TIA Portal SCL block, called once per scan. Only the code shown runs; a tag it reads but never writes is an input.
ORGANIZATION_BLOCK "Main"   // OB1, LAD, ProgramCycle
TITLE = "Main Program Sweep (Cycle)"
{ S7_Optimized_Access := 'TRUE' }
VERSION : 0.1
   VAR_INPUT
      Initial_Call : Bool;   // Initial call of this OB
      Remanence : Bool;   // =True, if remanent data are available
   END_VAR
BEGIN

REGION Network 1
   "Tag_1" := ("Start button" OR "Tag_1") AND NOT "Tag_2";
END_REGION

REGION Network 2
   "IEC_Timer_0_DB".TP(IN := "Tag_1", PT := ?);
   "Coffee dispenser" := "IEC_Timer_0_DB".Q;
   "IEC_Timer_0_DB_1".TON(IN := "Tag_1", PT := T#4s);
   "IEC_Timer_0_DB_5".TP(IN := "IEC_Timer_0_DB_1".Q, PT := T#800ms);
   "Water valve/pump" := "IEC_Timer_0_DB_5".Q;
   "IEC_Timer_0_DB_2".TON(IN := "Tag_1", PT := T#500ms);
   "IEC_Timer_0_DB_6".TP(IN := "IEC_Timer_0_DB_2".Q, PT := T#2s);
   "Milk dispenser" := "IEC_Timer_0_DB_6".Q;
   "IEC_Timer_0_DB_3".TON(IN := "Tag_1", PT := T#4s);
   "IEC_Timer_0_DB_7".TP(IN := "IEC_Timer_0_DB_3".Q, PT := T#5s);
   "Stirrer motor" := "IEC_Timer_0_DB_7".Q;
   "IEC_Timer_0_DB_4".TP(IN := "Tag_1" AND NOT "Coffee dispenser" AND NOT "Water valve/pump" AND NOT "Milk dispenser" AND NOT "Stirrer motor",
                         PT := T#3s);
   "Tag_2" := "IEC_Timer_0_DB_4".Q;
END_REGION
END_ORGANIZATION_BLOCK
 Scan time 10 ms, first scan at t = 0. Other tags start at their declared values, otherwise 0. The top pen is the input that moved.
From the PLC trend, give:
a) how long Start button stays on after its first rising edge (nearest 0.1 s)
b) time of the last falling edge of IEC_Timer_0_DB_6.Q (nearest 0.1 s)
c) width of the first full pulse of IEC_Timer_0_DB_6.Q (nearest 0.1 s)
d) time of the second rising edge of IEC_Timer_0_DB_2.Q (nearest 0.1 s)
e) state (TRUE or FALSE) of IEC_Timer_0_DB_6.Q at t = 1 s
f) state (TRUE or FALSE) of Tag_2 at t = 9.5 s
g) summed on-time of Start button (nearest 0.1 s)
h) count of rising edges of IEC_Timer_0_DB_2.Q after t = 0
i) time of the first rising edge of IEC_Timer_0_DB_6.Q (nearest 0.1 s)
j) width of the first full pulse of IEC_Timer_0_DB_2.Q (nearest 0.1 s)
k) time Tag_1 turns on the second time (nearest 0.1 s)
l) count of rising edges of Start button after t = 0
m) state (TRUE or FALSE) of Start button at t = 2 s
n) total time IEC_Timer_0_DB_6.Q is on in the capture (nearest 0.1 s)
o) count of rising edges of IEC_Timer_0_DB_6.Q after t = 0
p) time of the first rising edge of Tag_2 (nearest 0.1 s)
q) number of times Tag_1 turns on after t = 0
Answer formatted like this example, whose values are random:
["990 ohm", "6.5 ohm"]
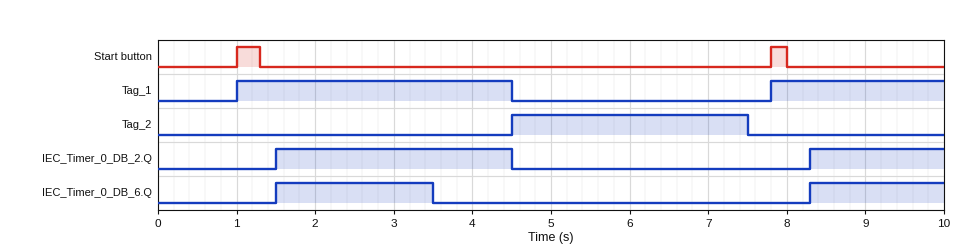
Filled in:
["0.3 s", "3.5 s", "2.0 s", "8.3 s", "FALSE", "FALSE", "0.5 s", "2", "1.5 s", "3.0 s", "7.8 s", "2", "FALSE", "3.7 s", "2", "4.5 s", "2"]
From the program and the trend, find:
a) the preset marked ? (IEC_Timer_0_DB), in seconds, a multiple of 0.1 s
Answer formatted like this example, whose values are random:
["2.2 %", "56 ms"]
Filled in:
["3.5 s"]
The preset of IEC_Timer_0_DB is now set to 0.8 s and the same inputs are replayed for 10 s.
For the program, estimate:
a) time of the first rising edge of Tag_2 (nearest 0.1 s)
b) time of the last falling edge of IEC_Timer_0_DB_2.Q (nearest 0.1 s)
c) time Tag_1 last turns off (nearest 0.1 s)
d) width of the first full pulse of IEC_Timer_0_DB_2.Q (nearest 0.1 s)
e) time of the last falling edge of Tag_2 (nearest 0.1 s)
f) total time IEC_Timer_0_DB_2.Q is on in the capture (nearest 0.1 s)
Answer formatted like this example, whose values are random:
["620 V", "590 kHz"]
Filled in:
["3.5 s", "3.5 s", "3.5 s", "2.0 s", "6.5 s", "3.7 s"]
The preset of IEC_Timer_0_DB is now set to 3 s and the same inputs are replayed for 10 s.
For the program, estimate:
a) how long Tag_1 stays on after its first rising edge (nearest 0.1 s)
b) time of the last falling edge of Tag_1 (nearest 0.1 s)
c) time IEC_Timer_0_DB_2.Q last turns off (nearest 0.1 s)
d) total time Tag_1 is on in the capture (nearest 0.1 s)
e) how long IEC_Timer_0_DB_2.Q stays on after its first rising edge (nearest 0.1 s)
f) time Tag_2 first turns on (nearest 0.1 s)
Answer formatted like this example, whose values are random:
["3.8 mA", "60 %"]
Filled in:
["3.0 s", "4.0 s", "4.0 s", "5.2 s", "2.5 s", "4.0 s"]
